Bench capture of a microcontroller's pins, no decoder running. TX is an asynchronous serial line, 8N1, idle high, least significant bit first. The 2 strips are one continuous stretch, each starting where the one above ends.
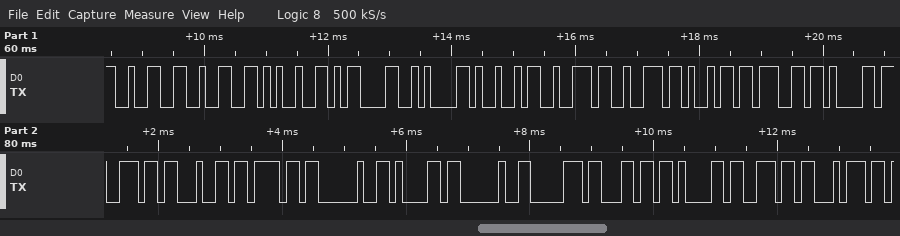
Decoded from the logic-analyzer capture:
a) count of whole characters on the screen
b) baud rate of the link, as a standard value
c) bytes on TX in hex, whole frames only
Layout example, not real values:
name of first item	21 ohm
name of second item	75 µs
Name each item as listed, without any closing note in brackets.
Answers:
count of whole characters on the screen	22
baud rate of the link, as a standard value	9600 baud
bytes on TX in hex, whole frames only	32 32 25 0D 0A 49 72 72 69 67 61 6E 64 6F 20 61 20 70 6C 61 6E 74
